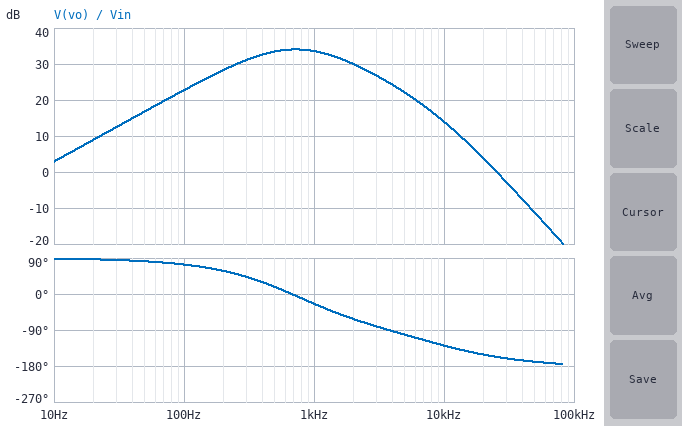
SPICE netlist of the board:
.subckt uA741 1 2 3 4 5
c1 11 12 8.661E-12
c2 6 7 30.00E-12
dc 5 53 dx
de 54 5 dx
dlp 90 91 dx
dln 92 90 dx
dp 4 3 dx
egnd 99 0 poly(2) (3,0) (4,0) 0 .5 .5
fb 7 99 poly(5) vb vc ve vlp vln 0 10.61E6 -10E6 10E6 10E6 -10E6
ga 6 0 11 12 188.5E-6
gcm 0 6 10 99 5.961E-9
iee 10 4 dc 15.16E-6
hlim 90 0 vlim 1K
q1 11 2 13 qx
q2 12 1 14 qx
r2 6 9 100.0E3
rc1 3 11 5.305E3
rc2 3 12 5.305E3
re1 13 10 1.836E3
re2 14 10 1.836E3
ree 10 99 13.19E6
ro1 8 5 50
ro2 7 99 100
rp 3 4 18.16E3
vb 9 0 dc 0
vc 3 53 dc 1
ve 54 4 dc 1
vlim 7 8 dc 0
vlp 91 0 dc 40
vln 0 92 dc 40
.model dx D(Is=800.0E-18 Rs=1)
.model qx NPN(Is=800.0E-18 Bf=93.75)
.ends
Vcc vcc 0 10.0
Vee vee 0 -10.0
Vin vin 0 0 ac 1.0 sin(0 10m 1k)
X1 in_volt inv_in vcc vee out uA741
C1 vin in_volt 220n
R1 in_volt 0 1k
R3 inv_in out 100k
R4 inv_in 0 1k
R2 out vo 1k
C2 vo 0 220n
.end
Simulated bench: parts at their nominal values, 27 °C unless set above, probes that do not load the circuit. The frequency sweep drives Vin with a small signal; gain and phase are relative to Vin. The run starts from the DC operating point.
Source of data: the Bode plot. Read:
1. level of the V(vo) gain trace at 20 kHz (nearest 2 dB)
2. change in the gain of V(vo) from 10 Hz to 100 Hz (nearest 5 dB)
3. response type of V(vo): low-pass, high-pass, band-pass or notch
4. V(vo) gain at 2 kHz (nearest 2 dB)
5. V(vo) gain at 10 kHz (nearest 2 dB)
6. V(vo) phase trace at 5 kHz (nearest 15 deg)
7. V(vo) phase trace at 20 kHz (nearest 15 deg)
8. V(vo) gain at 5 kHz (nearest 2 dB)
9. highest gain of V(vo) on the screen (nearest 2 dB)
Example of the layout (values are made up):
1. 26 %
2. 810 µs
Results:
1. 4 dB
2. 20 dB
3. band-pass
4. 30 dB
5. 14 dB
6. -105 deg
7. -150 deg
8. 22 dB
9. 34 dB
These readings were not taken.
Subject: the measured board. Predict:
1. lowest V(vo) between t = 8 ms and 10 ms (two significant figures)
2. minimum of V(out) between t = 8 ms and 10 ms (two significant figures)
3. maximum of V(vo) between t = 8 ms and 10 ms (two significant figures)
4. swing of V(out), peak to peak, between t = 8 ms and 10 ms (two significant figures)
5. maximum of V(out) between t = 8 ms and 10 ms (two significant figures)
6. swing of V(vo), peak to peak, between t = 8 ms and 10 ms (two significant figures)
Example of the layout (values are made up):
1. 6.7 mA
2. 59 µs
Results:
1. -480 mV
2. -810 mV
3. 480 mV
4. 1.6 V
5. 820 mV
6. 960 mV
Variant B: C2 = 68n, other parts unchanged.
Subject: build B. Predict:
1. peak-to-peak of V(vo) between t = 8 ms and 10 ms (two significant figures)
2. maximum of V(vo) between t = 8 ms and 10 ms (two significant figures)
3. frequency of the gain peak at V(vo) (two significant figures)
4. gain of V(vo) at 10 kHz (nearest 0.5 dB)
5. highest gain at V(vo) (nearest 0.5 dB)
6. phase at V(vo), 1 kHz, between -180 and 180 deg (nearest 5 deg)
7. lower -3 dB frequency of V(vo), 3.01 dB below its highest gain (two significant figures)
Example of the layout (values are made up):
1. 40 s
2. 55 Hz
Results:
1. 1.5 V
2. 750 mV
3. 1.3 kHz
4. 24.0 dB
5. 37.5 dB
6. 5 deg
7. 470 Hz
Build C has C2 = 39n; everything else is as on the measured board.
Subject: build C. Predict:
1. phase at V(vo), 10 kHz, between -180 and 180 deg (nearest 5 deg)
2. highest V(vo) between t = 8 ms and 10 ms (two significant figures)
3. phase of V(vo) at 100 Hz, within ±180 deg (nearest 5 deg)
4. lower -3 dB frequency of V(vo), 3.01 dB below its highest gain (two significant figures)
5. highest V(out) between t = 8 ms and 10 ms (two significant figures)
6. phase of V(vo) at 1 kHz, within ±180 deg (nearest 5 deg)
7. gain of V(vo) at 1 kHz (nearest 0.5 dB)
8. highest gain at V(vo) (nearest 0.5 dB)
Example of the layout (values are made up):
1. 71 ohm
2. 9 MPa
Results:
1. -110 deg
2. 790 mV
3. 80 deg
4. 540 Hz
5. 820 mV
6. 15 deg
7. 38.0 dB
8. 38.5 dB
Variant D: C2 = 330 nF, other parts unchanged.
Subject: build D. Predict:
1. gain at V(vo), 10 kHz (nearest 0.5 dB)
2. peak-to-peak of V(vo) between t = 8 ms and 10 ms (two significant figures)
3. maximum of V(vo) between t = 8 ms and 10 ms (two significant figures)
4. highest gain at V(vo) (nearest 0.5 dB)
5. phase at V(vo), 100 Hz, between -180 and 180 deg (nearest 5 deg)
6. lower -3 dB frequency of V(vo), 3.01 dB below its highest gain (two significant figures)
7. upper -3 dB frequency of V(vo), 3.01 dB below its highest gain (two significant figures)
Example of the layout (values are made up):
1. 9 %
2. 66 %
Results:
1. 10.5 dB
2. 710 mV
3. 360 mV
4. 32.0 dB
5. 70 deg
6. 240 Hz
7. 1.4 kHz
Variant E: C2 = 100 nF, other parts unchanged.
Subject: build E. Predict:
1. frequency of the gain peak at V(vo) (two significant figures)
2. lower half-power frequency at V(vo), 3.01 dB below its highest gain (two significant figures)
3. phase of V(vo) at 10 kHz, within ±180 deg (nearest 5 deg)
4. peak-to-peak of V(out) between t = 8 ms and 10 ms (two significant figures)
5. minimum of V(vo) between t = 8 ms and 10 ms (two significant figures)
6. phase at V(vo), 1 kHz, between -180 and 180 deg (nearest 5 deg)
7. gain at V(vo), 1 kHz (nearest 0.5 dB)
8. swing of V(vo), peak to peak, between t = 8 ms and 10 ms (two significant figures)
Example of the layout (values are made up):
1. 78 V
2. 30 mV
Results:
1. 1.1 kHz
2. 420 Hz
3. -125 deg
4. 1.6 V
5. -690 mV
6. 0 deg
7. 37.0 dB
8. 1.4 V
